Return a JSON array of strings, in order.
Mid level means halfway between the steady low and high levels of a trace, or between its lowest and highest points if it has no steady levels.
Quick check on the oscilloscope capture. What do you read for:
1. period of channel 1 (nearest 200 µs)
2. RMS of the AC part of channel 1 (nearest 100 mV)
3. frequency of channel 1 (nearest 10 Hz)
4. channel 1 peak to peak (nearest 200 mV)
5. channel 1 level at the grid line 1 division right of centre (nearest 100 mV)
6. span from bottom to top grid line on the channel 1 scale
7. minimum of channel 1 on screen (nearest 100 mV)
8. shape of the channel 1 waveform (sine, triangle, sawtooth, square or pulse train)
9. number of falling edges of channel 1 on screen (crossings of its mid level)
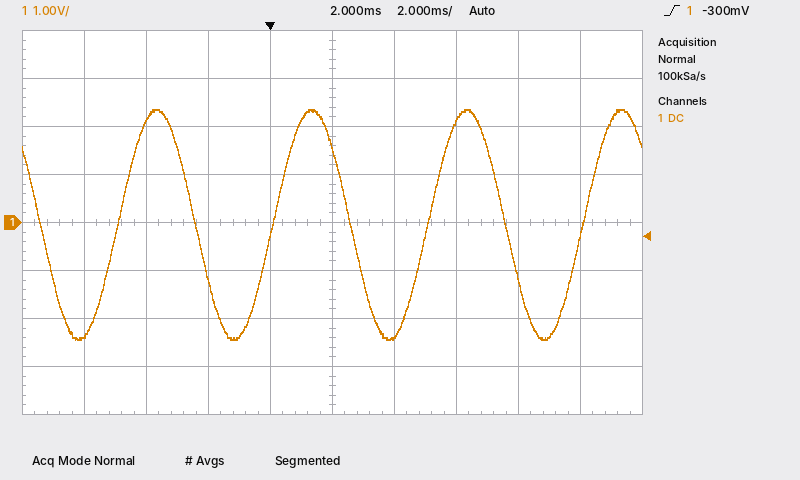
["5.0 ms", "1.7 V", "200 Hz", "4.8 V", "-2.4 V", "8 V", "-2.4 V", "sine", "4"]
